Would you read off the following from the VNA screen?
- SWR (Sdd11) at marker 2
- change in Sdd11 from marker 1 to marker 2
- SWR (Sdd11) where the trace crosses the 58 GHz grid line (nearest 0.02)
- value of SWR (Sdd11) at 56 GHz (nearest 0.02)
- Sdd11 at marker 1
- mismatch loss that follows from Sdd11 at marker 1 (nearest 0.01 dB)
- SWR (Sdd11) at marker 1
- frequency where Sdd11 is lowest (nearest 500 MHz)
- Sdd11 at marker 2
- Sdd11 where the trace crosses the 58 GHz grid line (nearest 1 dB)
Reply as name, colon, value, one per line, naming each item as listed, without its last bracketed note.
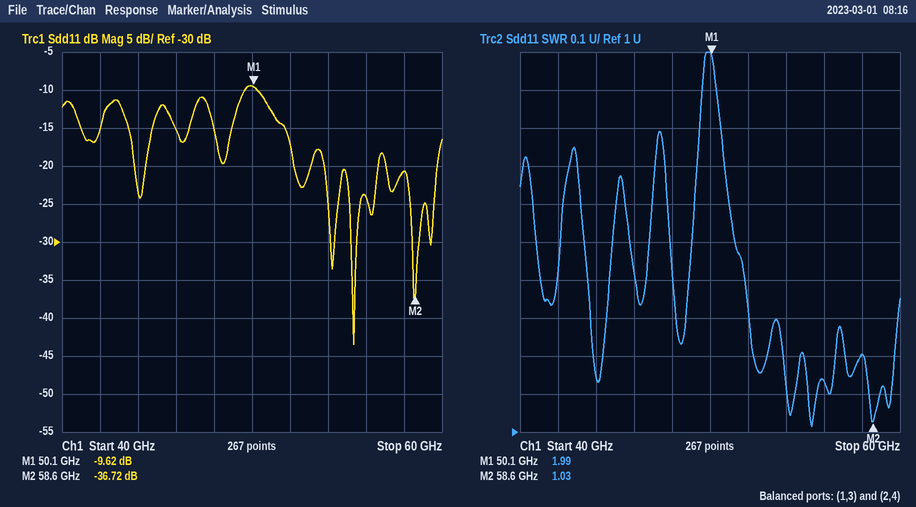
SWR (Sdd11) at marker 2: 1.03
change in Sdd11 from marker 1 to marker 2: -27.10 dB
SWR (Sdd11) where the trace crosses the 58 GHz grid line: 1.20
value of SWR (Sdd11) at 56 GHz: 1.14
Sdd11 at marker 1: -9.62 dB
mismatch loss that follows from Sdd11 at marker 1: 0.50 dB
SWR (Sdd11) at marker 1: 1.99
frequency where Sdd11 is lowest: 55.5 GHz
Sdd11 at marker 2: -36.72 dB
Sdd11 where the trace crosses the 58 GHz grid line: -21 dB
